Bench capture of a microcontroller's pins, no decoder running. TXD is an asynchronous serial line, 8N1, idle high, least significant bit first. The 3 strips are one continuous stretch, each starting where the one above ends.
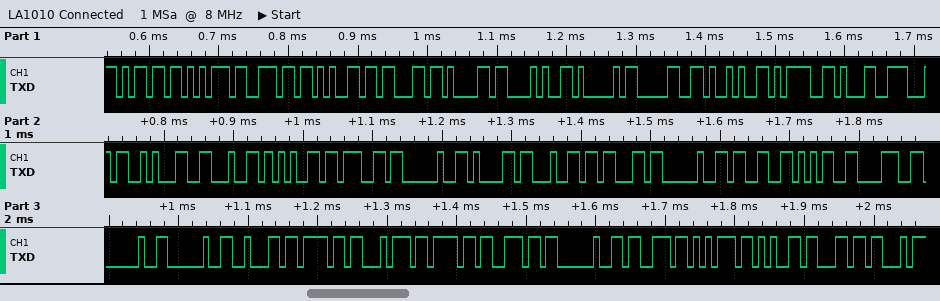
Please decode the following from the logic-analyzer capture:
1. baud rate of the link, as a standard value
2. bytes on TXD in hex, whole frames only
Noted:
115200 baud
0x6D 0x75 0x6E 0x65 0x63 0x61 0x28 0x41 0x30 0x29 0x3D 0x31 0x34 0x31 0x64 0x65 0x67 0x20 0x61 0x64 0x63 0x20 0x33 0x35 0x38 0x20 0x20 0x62 0x6F 0x74 0x6F 0x6E 0x20 0x73 0x75 0x65 0x6C
